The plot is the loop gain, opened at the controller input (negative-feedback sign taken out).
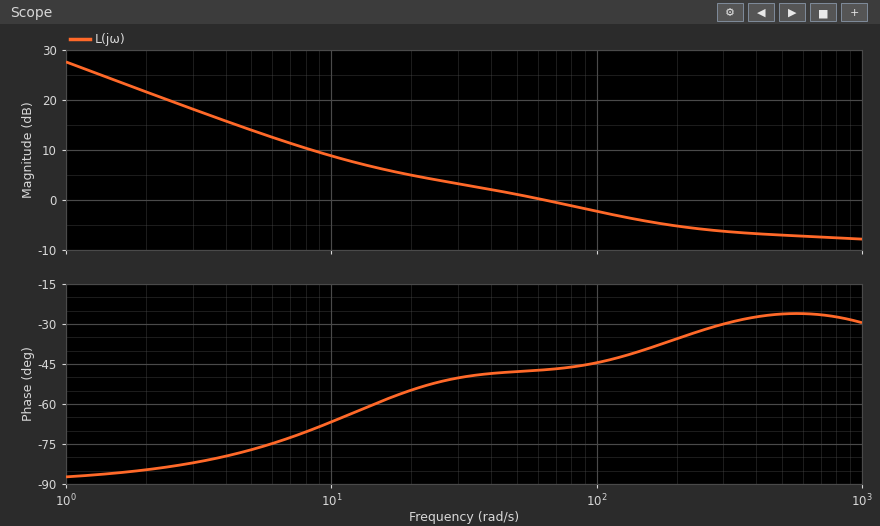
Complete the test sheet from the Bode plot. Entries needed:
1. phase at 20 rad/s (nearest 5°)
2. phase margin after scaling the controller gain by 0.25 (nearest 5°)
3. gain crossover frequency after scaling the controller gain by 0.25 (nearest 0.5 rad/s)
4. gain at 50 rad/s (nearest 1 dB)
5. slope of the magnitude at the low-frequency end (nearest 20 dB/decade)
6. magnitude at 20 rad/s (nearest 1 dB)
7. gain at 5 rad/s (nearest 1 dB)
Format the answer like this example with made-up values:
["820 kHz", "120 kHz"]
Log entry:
["-55°", "105°", "6.5 rad/s", "1 dB", "-20 dB/decade", "5 dB", "14 dB"]
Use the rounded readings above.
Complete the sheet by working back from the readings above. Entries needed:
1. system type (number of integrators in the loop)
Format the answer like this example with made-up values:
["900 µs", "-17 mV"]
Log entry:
["1"]
